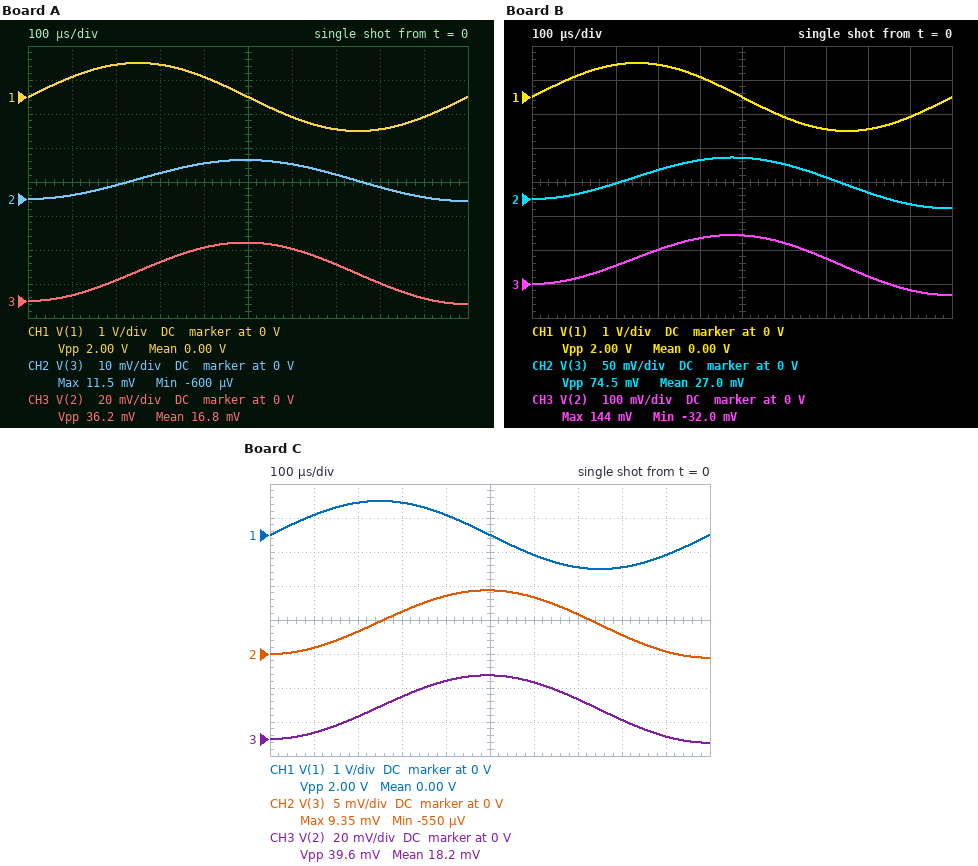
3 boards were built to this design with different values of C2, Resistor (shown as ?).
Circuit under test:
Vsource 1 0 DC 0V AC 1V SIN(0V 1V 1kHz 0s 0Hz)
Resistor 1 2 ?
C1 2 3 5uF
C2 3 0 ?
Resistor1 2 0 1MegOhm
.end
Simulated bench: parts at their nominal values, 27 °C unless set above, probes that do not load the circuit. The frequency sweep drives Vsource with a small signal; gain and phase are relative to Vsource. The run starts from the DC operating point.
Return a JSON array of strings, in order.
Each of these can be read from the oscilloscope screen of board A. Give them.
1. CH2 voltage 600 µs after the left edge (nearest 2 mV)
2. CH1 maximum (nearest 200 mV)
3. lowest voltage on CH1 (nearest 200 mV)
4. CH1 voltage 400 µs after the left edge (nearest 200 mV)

["10 mV", "1.0 V", "-1.0 V", "600 mV"]
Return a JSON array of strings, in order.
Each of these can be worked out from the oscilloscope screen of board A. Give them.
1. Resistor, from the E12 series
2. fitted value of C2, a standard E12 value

["2.7 kΩ", "10 µF"]
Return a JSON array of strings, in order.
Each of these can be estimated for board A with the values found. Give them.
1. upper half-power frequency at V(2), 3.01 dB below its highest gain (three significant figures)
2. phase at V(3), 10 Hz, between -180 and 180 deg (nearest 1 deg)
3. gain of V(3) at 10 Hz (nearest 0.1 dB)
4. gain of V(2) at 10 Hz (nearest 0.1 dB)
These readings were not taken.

["17.7 Hz", "-29 deg", "-10.8 dB", "-1.2 dB"]
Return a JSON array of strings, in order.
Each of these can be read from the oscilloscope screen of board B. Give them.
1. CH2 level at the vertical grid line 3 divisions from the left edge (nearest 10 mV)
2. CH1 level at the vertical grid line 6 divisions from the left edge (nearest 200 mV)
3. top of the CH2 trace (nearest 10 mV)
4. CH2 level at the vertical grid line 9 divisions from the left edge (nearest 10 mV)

["40 mV", "-600 mV", "60 mV", "-10 mV"]
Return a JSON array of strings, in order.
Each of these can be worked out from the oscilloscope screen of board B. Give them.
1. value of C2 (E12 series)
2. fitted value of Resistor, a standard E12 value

["6.8 µF", "680 Ω"]
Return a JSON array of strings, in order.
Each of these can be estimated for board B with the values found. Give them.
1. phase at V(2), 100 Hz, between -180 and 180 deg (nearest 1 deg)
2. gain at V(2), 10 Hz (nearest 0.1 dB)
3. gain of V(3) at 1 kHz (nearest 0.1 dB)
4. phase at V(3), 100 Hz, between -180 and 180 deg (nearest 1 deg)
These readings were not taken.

["-51 deg", "-0.1 dB", "-29.3 dB", "-51 deg"]
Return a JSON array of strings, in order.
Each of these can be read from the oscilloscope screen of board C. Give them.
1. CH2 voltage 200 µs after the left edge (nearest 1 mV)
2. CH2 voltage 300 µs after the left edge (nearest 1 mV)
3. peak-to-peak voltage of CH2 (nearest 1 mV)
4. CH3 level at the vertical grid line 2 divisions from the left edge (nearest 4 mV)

["3 mV", "6 mV", "10 mV", "12 mV"]
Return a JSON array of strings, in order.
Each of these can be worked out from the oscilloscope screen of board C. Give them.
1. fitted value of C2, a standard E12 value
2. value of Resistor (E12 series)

["15 µF", "2.2 kΩ"]
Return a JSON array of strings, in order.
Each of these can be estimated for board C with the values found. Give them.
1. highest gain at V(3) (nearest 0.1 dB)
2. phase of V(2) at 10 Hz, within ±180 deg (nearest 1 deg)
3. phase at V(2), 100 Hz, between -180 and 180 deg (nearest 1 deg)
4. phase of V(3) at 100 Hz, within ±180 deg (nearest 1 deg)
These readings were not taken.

["-12.1 dB", "-27 deg", "-79 deg", "-79 deg"]
